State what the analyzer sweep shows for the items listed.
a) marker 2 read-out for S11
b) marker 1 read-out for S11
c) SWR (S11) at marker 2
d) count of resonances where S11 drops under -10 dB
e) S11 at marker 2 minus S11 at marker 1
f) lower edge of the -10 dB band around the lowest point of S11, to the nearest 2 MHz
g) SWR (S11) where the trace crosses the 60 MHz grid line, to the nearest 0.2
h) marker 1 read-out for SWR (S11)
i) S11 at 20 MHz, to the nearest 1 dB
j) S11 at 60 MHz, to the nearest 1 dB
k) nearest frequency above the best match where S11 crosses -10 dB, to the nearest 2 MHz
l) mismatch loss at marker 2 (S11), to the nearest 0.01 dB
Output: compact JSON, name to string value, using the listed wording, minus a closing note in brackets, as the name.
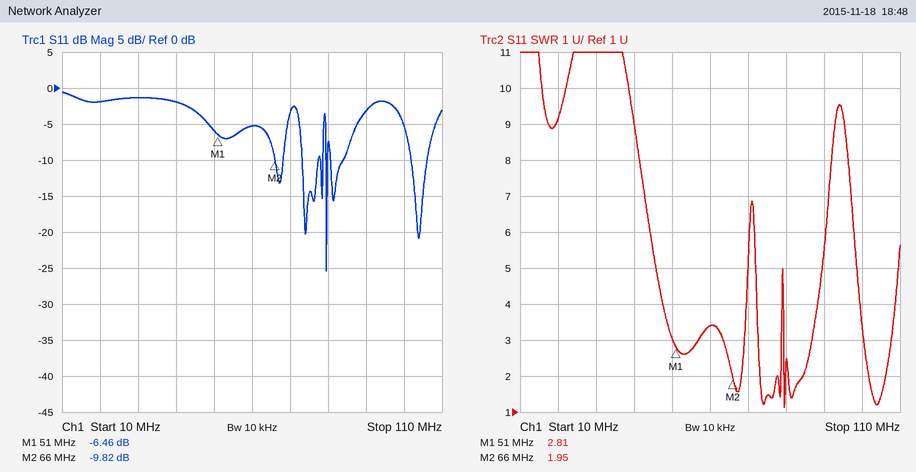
{"marker 2 read-out for S11": "-9.82 dB", "marker 1 read-out for S11": "-6.46 dB", "SWR (S11) at marker 2": "1.95", "count of resonances where S11 drops under -10 dB": "6", "S11 at marker 2 minus S11 at marker 1": "-3.36 dB", "lower edge of the -10 dB band around the lowest point of S11, to the nearest 2 MHz": "80 MHz", "SWR (S11) where the trace crosses the 60 MHz grid line, to the nearest 0.2": "3.4", "marker 1 read-out for SWR": "2.81", "S11 at 20 MHz, to the nearest 1 dB": "-2 dB", "S11 at 60 MHz, to the nearest 1 dB": "-5 dB", "nearest frequency above the best match where S11 crosses -10 dB, to the nearest 2 MHz": "80 MHz", "mismatch loss at marker 2 (S11), to the nearest 0.01 dB": "0.48 dB"}
